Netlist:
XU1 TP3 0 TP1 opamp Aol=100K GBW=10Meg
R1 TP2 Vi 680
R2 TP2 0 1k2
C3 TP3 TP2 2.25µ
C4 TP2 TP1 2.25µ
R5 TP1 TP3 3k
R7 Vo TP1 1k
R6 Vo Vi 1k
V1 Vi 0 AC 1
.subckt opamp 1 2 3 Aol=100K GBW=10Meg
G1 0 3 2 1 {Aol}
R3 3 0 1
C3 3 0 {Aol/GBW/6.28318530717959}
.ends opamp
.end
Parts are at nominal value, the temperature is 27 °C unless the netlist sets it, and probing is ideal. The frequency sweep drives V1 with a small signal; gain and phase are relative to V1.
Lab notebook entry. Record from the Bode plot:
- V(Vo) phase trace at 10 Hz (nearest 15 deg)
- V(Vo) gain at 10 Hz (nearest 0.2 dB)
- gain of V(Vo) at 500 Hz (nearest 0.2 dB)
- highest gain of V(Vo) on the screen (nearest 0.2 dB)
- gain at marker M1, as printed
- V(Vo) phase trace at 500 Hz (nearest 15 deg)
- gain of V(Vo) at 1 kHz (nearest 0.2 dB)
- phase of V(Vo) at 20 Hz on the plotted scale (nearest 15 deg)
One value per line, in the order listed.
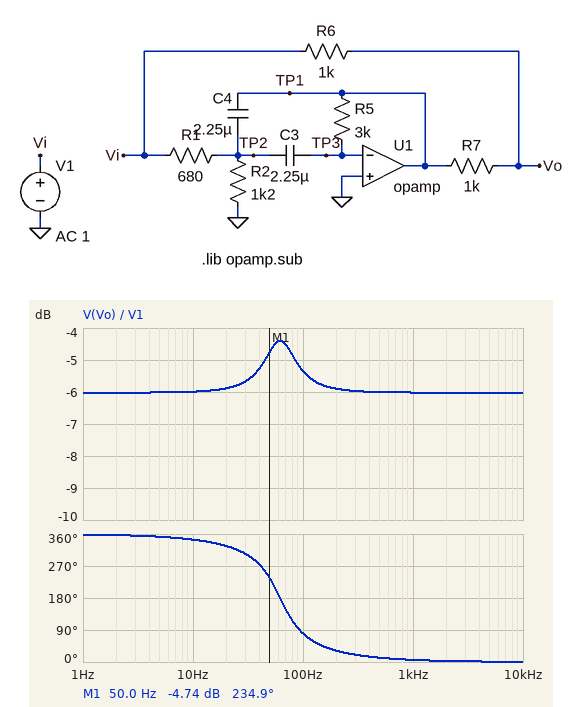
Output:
345 deg
-6.0 dB
-6.0 dB
-4.4 dB
-4.74 dB
15 deg
-6.0 dB
330 deg
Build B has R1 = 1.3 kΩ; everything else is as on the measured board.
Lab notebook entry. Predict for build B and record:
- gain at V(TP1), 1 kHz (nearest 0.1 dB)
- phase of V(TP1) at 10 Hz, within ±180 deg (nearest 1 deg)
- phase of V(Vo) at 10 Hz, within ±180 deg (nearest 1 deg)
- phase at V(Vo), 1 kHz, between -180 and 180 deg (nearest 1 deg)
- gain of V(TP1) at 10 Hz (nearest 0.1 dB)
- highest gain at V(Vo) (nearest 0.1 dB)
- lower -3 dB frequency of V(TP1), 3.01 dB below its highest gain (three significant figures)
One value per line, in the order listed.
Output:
-25.3 dB
-100 deg
-12 deg
3 deg
-13.6 dB
-6.0 dB
33.2 Hz
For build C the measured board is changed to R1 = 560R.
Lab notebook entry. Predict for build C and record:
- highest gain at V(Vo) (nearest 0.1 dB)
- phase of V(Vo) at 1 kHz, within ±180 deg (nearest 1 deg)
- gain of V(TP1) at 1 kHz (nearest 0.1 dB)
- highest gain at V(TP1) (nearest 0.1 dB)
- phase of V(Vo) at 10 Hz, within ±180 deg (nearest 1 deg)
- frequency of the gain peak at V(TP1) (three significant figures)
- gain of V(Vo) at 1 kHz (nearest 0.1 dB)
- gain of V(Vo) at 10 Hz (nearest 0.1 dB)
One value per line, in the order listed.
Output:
-1.5 dB
7 deg
-17.9 dB
8.6 dB
-17 deg
66.1 Hz
-6.0 dB
-5.9 dB
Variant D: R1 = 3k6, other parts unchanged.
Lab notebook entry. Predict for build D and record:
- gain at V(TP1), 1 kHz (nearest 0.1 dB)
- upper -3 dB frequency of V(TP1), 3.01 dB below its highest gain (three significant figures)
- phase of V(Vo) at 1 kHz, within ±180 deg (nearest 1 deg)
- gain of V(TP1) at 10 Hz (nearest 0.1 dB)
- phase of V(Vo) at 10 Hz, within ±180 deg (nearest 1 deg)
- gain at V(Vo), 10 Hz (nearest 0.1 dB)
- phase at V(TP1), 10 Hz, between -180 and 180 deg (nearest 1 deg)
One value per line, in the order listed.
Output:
-34.1 dB
72.7 Hz
1 deg
-19.3 dB
-6 deg
-6.2 dB
-105 deg
